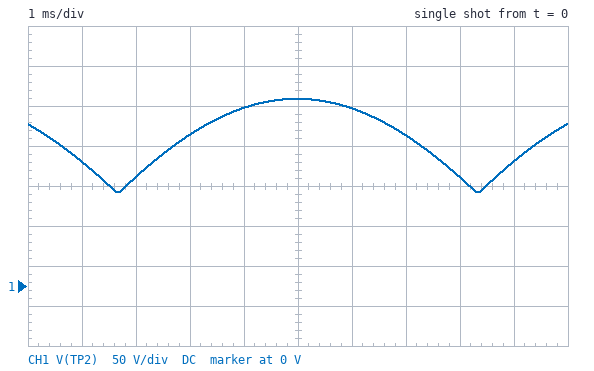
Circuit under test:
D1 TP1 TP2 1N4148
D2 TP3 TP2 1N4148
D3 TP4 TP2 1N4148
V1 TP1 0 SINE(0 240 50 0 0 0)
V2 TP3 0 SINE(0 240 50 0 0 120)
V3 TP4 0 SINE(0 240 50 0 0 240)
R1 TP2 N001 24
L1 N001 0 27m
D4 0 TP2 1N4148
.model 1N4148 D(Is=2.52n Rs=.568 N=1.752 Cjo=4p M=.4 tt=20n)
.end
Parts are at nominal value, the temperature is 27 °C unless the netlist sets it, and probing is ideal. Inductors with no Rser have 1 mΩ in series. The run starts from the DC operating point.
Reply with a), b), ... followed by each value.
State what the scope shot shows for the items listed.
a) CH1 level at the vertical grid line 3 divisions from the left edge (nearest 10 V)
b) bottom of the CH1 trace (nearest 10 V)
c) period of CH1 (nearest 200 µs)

a) 190 V
b) 120 V
c) 6.6 ms
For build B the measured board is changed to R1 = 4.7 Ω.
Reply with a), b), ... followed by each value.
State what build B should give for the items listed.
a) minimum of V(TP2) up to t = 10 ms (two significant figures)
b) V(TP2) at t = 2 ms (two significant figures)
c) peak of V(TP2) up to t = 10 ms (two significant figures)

a) 110 V
b) 120 V
c) 220 V
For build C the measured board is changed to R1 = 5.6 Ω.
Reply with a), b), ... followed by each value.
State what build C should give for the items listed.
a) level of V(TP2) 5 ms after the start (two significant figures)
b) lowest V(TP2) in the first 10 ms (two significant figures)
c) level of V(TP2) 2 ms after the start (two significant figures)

a) 220 V
b) 110 V
c) 120 V
